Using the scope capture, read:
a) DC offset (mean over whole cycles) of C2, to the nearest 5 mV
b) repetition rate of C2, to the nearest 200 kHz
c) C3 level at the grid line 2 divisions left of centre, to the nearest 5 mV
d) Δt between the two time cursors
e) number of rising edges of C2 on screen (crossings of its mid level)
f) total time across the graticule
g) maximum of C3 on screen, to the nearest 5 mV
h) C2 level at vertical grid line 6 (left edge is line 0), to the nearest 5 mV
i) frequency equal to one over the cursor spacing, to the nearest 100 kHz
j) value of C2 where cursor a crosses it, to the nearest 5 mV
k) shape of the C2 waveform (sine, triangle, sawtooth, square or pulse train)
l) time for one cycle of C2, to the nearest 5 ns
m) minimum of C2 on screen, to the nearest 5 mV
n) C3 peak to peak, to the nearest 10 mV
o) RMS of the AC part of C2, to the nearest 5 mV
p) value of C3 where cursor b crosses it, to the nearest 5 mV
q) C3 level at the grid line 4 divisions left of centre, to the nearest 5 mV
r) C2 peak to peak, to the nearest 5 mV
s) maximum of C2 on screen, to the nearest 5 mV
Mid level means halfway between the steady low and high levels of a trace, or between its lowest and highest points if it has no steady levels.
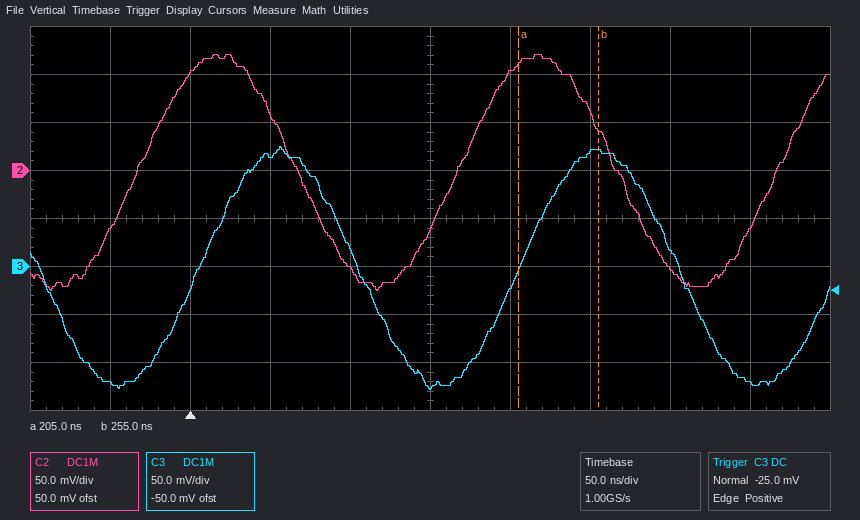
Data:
0 mV
5.0 MHz
115 mV
50 ns
3
500 ns
125 mV
100 mV
20.0 MHz
110 mV
sine
200 ns
-125 mV
250 mV
85 mV
120 mV
-120 mV
245 mV
120 mV
